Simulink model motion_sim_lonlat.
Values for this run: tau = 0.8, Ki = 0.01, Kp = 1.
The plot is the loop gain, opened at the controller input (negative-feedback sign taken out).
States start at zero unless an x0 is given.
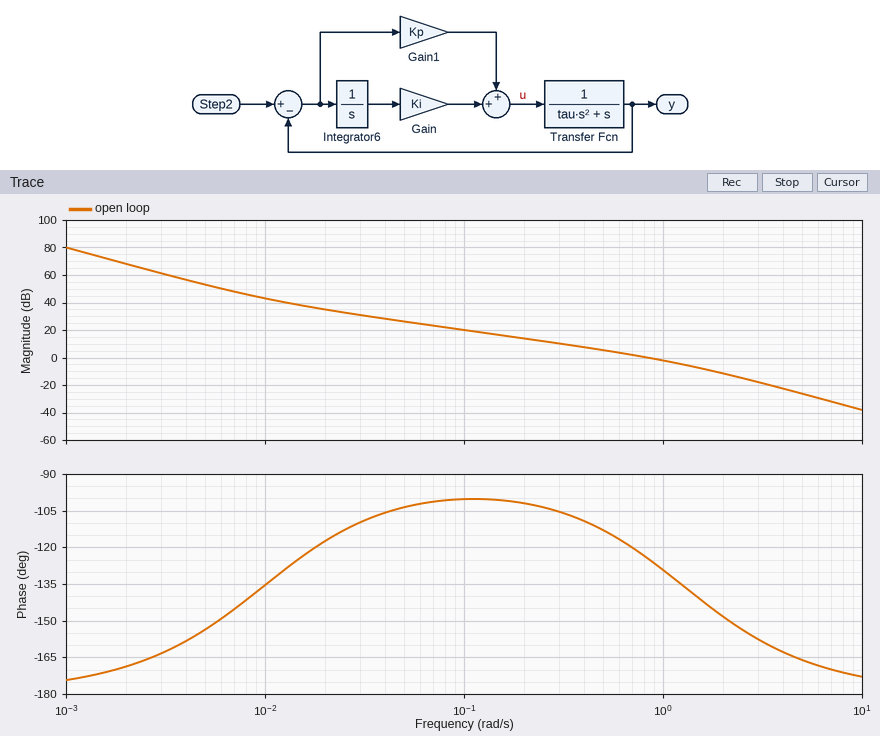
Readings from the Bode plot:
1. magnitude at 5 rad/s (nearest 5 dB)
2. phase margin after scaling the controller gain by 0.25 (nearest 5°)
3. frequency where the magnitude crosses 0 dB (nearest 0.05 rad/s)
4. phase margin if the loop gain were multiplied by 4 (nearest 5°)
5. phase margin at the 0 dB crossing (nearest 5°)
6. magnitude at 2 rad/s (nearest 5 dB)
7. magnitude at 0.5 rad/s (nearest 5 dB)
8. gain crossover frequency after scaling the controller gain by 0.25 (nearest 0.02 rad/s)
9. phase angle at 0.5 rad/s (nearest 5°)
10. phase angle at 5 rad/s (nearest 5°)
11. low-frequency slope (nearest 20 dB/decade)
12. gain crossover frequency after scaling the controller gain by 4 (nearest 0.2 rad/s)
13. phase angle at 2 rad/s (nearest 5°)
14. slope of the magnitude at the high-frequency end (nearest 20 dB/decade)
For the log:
-25 dB
75°
0.85 rad/s
30°
55°
-10 dB
5 dB
0.24 rad/s
-115°
-165°
-40 dB/decade
2.0 rad/s
-150°
-40 dB/decade
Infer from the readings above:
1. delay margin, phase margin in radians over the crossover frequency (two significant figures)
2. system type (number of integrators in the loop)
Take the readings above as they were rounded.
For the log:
1.1 s
2
